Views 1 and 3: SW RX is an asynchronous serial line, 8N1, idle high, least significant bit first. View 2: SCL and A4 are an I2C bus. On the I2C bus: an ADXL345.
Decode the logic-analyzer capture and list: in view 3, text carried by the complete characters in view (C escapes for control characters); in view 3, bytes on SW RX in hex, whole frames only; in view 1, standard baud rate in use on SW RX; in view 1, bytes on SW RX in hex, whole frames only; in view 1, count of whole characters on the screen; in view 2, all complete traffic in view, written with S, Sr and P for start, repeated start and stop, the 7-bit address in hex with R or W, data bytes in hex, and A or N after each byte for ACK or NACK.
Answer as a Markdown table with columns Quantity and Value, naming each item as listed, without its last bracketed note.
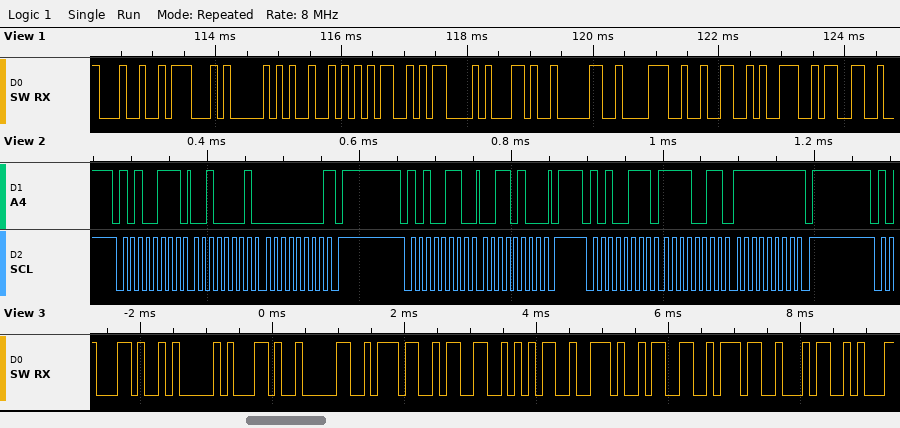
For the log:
| Quantity | Value |
|---|---|
| in view 3, text carried by the complete characters in view | ",A,0735.374" |
| in view 3, bytes on SW RX in hex, whole frames only | 2C 41 2C 30 37 33 35 2E 33 37 34 |
| in view 1, standard baud rate in use on SW RX | 9600 baud |
| in view 1, bytes on SW RX in hex, whole frames only | 0x24 0x47 0x50 0x52 0x4D 0x43 0x2C 0x30 0x38 0x32 0x39 0x33 |
| in view 1, count of whole characters on the screen | 12 |
| in view 2, all complete traffic in view, written with S, Sr and P for start, repeated start and stop, the 7-bit address in hex with R or W, data bytes in hex, and A or N after each byte for ACK or NACK | S 53R A 21 A 00 N P S 53W A 34 A P S 53R A F3 A FF N P |
